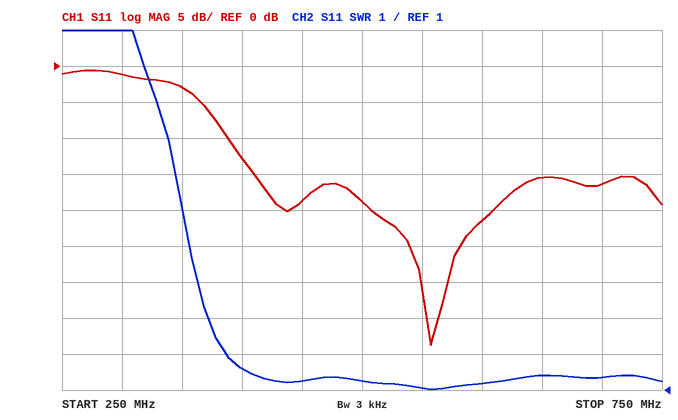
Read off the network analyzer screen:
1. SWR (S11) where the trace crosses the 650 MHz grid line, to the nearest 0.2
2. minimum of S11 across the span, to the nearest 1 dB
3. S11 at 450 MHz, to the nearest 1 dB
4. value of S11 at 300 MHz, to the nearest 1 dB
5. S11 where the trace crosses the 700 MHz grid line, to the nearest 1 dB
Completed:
1.4
-39 dB
-19 dB
-1 dB
-16 dB
